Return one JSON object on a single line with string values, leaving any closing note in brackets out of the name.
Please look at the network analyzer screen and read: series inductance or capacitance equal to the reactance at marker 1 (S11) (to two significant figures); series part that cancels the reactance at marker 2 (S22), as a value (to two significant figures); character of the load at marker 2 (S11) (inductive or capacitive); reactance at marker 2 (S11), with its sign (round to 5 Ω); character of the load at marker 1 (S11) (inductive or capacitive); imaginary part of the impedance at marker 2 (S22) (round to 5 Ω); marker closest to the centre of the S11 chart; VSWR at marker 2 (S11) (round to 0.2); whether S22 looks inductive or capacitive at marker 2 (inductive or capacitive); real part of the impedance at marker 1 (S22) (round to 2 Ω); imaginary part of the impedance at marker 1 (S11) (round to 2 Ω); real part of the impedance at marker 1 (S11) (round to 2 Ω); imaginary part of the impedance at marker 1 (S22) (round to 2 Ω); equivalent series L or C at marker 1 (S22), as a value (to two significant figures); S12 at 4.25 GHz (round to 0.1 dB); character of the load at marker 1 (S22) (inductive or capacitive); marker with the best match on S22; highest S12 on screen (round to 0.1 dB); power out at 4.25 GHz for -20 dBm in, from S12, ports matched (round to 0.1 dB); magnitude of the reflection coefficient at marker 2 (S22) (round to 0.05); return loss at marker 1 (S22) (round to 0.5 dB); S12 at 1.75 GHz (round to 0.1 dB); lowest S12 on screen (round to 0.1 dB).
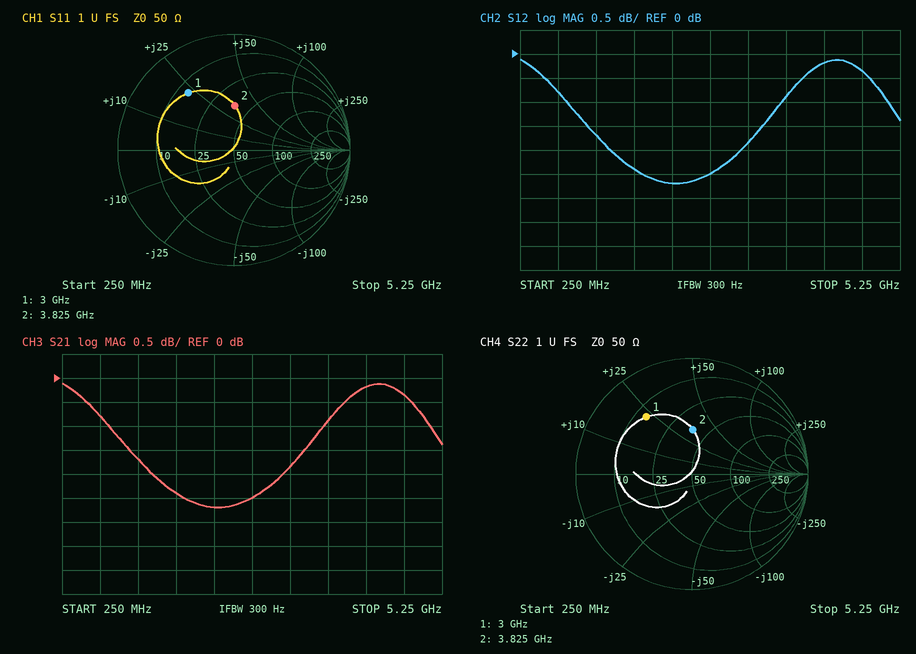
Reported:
{"series inductance or capacitance equal to the reactance at marker 1 (S11)": "1.2 nH", "series part that cancels the reactance at marker 2 (S22), as a value": "1.2 pF", "character of the load at marker 2 (S11)": "inductive", "reactance at marker 2 (S11), with its sign": "+35 Ω", "character of the load at marker 1 (S11)": "inductive", "imaginary part of the impedance at marker 2 (S22)": "+35 Ω", "marker closest to the centre of the S11 chart": "marker 2", "VSWR at marker 2 (S11)": "2.2", "whether S22 looks inductive or capacitive at marker 2": "inductive", "real part of the impedance at marker 1 (S22)": "14 Ω", "imaginary part of the impedance at marker 1 (S11)": "+22 Ω", "real part of the impedance at marker 1 (S11)": "14 Ω", "imaginary part of the impedance at marker 1 (S22)": "+22 Ω", "equivalent series L or C at marker 1 (S22), as a value": "1.2 nH", "S12 at 4.25 GHz": "-0.2 dB", "character of the load at marker 1 (S22)": "inductive", "marker with the best match on S22": "marker 2", "highest S12 on screen": "-0.1 dB", "power out at 4.25 GHz for -20 dBm in, from S12, ports matched": "-20.2 dBm", "magnitude of the reflection coefficient at marker 2 (S22)": "0.40", "return loss at marker 1 (S22)": "4.0 dB", "S12 at 1.75 GHz": "-2.4 dB", "lowest S12 on screen": "-2.7 dB"}
